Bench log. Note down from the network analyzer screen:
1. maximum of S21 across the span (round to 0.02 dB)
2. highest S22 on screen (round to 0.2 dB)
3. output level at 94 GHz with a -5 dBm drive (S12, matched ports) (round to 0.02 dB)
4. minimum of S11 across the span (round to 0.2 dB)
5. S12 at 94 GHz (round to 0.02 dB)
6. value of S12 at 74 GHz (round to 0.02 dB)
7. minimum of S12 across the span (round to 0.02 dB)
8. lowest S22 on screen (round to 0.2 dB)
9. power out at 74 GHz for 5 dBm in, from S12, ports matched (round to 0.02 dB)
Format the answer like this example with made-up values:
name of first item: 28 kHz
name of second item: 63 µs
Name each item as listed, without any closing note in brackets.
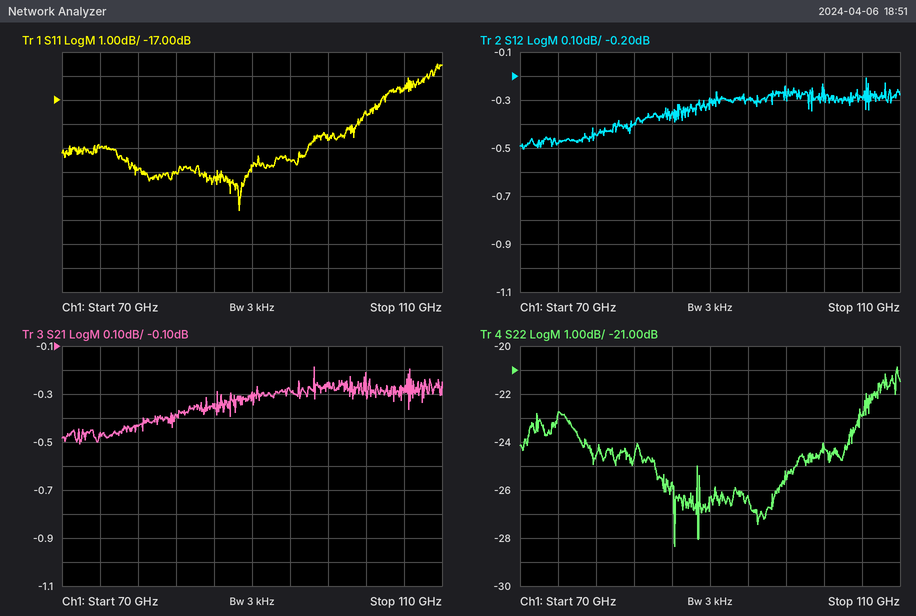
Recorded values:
maximum of S21 across the span: -0.18 dB
highest S22 on screen: -20.8 dB
output level at 94 GHz with a -5 dBm drive (S12, matched ports): -5.30 dBm
minimum of S11 across the span: -21.6 dB
S12 at 94 GHz: -0.30 dB
value of S12 at 74 GHz: -0.48 dB
minimum of S12 across the span: -0.50 dB
lowest S22 on screen: -28.4 dB
power out at 74 GHz for 5 dBm in, from S12, ports matched: 4.52 dBm
